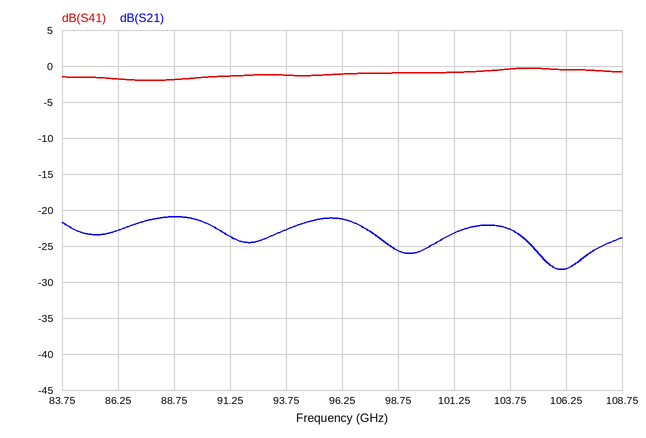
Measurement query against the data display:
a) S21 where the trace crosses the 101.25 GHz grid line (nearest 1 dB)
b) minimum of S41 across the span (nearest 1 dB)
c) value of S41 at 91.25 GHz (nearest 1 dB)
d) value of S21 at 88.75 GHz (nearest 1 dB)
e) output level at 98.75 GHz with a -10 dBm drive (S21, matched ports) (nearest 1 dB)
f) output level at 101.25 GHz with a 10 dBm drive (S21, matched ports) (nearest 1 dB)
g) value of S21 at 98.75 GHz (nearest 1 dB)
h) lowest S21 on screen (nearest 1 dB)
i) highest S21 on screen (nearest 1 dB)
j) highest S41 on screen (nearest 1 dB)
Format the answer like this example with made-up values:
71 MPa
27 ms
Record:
-23 dB
-2 dB
-1 dB
-21 dB
-36 dBm
-13 dBm
-26 dB
-28 dB
-21 dB
0 dB
